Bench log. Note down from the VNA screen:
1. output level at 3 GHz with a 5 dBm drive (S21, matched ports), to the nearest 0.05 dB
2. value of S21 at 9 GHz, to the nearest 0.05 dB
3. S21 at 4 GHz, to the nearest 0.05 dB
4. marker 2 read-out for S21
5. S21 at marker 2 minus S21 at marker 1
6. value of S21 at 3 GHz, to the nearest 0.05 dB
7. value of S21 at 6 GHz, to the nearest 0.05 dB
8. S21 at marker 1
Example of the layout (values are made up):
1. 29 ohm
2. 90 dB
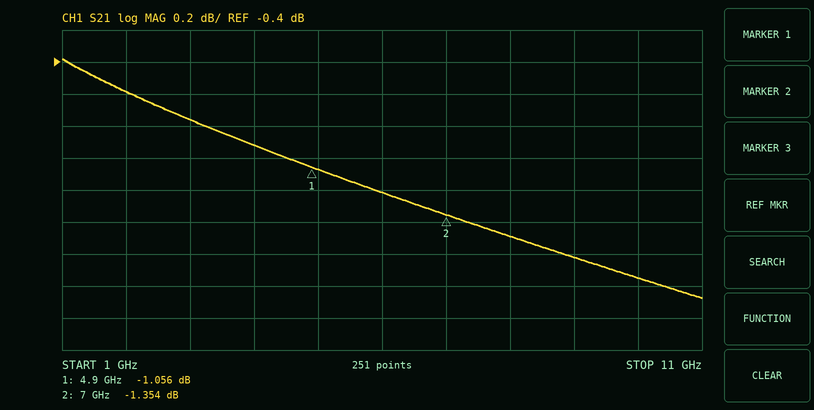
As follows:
1. 4.25 dBm
2. -1.60 dB
3. -0.90 dB
4. -1.354 dB
5. -0.298 dB
6. -0.75 dB
7. -1.20 dB
8. -1.056 dB
